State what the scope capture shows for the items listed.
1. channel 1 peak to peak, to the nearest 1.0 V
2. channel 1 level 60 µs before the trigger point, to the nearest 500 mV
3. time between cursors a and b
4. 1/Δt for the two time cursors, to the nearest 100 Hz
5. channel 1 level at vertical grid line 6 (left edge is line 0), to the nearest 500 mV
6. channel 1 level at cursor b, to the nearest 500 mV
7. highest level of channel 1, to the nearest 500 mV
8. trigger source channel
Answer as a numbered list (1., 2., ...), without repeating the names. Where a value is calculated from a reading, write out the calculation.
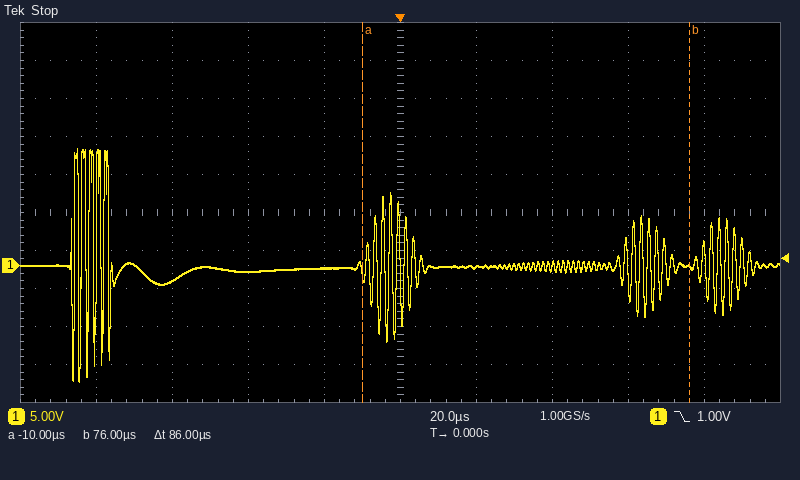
1. 31.0 V
2. -2.0 V
3. 86 µs
4. 1 / 86 µs ≈ 11.6 kHz
5. 0.0 V
6. 0.0 V
7. 15.5 V
8. channel 1
